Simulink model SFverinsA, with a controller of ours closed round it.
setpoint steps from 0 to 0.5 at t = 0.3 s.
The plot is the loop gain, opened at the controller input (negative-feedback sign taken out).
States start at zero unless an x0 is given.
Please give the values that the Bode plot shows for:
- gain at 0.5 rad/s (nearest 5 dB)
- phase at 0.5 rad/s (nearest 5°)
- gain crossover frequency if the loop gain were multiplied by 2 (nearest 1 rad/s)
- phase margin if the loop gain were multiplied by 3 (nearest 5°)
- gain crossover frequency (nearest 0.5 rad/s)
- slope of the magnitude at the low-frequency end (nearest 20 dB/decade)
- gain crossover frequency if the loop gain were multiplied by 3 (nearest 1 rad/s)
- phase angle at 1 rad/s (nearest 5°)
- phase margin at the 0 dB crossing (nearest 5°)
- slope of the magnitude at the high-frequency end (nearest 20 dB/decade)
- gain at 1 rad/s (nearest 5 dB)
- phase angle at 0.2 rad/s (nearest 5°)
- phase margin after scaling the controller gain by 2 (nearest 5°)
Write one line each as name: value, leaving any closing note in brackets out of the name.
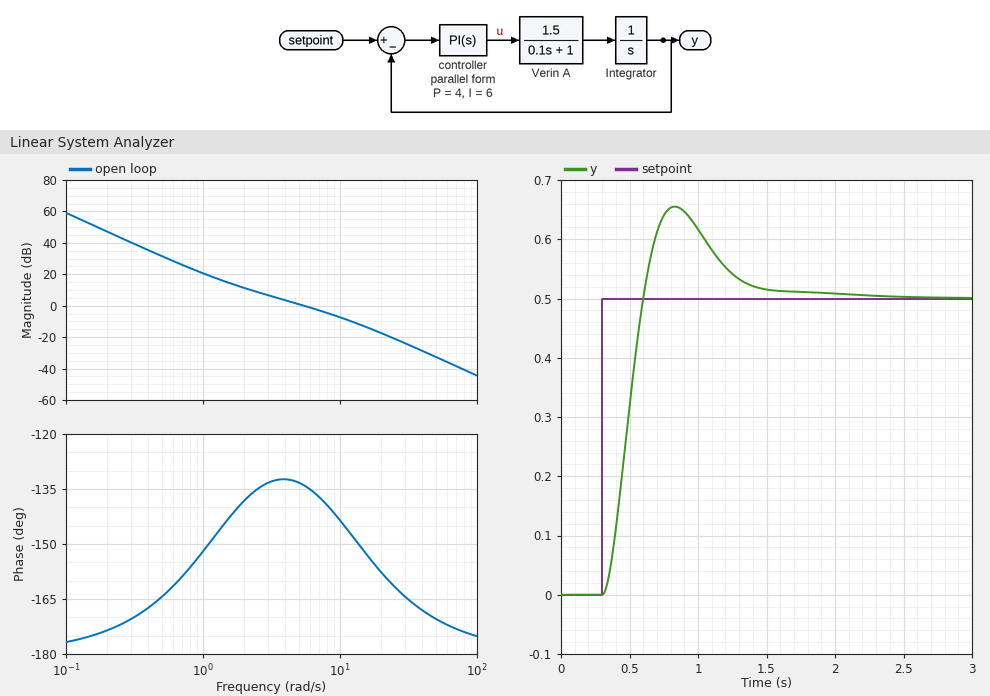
gain at 0.5 rad/s: 30 dB
phase at 0.5 rad/s: -165°
gain crossover frequency if the loop gain were multiplied by 2: 9 rad/s
phase margin if the loop gain were multiplied by 3: 35°
gain crossover frequency: 5.5 rad/s
slope of the magnitude at the low-frequency end: -40 dB/decade
gain crossover frequency if the loop gain were multiplied by 3: 12 rad/s
phase angle at 1 rad/s: -150°
phase margin at the 0 dB crossing: 45°
slope of the magnitude at the high-frequency end: -40 dB/decade
gain at 1 rad/s: 20 dB
phase angle at 0.2 rad/s: -175°
phase margin after scaling the controller gain by 2: 40°
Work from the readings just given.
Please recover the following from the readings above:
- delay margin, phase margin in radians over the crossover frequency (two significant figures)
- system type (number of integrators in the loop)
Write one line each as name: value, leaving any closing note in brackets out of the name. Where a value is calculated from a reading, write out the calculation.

delay margin, phase margin in radians over the crossover frequency: 45 × π / 180 / 5.5 = 0.14 s
system type: 2
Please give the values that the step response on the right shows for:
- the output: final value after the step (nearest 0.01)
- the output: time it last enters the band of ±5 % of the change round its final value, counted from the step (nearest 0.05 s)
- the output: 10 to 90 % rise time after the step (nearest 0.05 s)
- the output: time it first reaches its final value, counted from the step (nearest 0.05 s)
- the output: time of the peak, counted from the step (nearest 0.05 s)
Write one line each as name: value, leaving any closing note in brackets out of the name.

the output: final value after the step: 0.50
the output: time it last enters the band of ±5 % of the change round its final value, counted from the step: 1.05 s
the output: 10 to 90 % rise time after the step: 0.20 s
the output: time it first reaches its final value, counted from the step: 0.30 s
the output: time of the peak, counted from the step: 0.55 s
